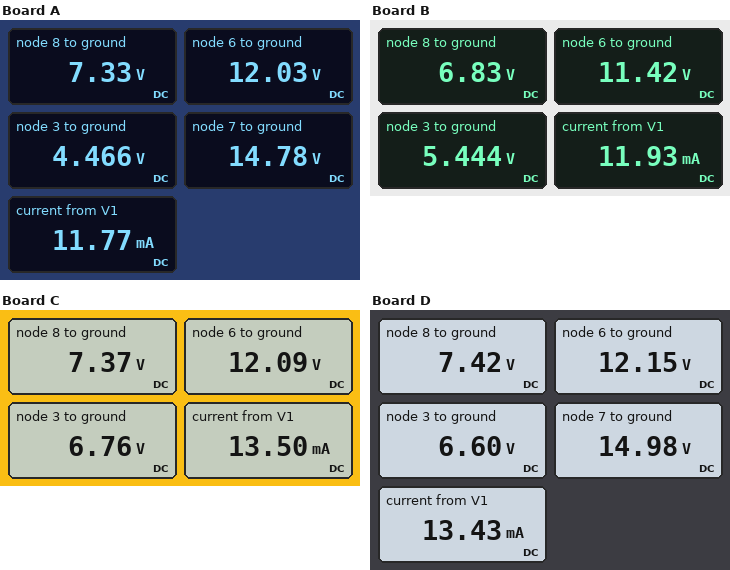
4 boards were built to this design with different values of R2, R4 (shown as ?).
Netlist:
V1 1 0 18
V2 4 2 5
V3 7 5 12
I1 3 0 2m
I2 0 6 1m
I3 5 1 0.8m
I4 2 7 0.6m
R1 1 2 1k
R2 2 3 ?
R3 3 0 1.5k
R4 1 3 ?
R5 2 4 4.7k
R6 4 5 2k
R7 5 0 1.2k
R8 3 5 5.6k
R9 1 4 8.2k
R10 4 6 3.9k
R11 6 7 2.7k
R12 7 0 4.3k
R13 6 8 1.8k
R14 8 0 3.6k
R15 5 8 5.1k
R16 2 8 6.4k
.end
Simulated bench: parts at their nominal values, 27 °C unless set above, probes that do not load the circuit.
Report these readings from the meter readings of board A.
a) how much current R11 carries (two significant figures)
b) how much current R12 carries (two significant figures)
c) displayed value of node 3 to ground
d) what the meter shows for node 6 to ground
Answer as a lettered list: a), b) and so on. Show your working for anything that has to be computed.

a) (14.78 V - 12.03 V) / 2.7 kΩ = 1.0 mA
b) (14.78 V) / 4.3 kΩ = 3.4 mA
c) 4.466 V
d) 12.03 V
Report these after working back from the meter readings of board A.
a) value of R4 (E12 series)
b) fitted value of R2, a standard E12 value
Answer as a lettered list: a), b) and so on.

a) 3.9 kΩ
b) 2.7 kΩ
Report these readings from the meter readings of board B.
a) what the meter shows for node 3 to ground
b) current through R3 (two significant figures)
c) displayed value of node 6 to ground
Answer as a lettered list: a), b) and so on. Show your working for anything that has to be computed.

a) 5.444 V
b) (5.444 V) / 1.5 kΩ = 3.6 mA
c) 11.42 V
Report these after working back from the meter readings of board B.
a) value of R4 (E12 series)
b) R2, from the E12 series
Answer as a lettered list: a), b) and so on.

a) 5.6 kΩ
b) 680 Ω
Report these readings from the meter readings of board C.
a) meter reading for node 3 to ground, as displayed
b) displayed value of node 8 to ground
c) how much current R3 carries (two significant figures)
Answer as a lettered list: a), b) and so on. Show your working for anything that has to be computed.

a) 6.76 V
b) 7.37 V
c) (6.76 V) / 1.5 kΩ = 4.5 mA
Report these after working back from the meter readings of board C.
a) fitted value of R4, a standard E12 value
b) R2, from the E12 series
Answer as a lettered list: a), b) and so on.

a) 2.2 kΩ
b) 1.2 kΩ
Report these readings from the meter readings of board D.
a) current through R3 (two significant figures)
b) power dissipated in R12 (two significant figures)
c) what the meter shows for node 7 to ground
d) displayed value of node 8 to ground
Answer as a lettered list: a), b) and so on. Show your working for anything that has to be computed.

a) (6.6 V) / 1.5 kΩ = 4.4 mA
b) (14.98 V)^2 / 4.3 kΩ = 52 mW
c) 14.98 V
d) 7.42 V
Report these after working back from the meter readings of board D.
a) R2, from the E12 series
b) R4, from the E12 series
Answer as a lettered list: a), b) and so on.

a) 1.5 kΩ
b) 2.2 kΩ
